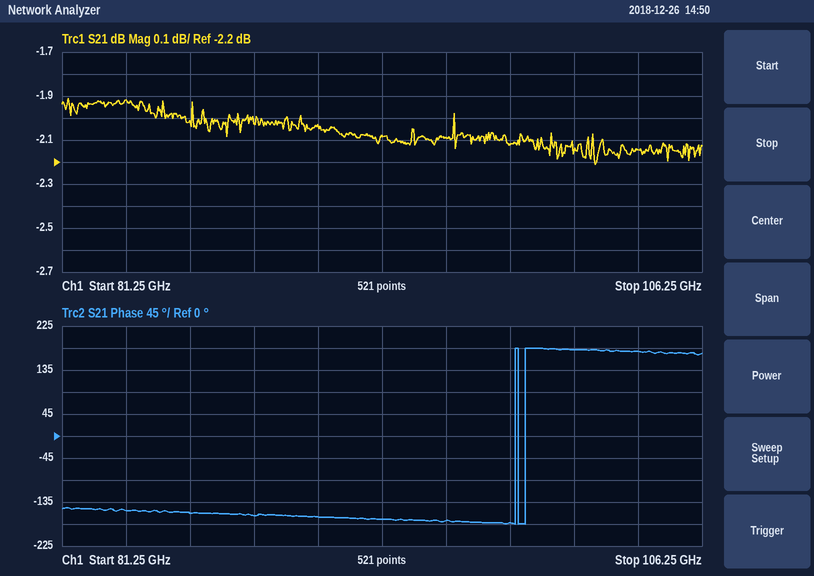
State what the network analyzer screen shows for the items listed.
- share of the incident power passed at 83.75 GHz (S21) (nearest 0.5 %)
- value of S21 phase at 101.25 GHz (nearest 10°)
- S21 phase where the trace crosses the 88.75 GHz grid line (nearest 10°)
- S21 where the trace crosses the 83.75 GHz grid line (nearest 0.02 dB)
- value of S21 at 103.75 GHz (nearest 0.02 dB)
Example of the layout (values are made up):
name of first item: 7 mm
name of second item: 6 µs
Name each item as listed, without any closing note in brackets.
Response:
share of the incident power passed at 83.75 GHz (S21): 64.5 %
value of S21 phase at 101.25 GHz: 180°
S21 phase where the trace crosses the 88.75 GHz grid line: -160°
S21 where the trace crosses the 83.75 GHz grid line: -1.92 dB
value of S21 at 103.75 GHz: -2.14 dB
